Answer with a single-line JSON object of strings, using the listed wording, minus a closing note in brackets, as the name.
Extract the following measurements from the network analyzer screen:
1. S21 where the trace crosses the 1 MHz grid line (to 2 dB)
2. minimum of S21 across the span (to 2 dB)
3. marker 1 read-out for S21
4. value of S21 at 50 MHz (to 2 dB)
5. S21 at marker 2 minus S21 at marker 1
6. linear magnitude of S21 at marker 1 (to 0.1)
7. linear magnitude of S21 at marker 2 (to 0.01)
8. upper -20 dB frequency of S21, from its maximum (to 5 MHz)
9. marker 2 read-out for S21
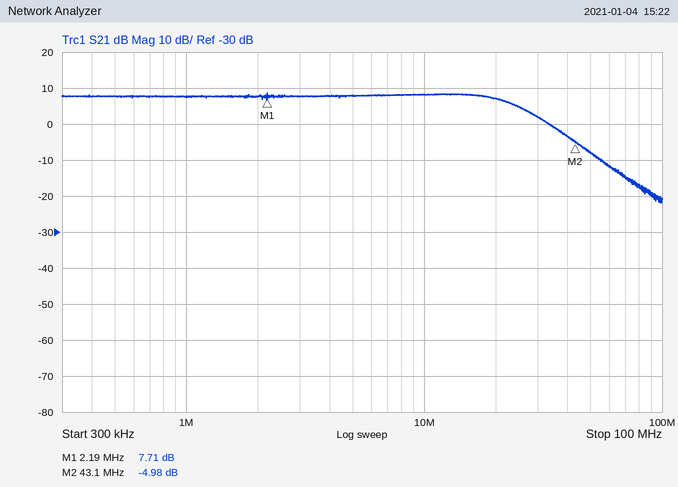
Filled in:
{"S21 where the trace crosses the 1 MHz grid line": "8 dB", "minimum of S21 across the span": "-22 dB", "marker 1 read-out for S21": "7.71 dB", "value of S21 at 50 MHz": "-8 dB", "S21 at marker 2 minus S21 at marker 1": "-12.69 dB", "linear magnitude of S21 at marker 1": "2.4", "linear magnitude of S21 at marker 2": "0.56", "upper -20 dB frequency of S21, from its maximum": "60 MHz", "marker 2 read-out for S21": "-4.98 dB"}
